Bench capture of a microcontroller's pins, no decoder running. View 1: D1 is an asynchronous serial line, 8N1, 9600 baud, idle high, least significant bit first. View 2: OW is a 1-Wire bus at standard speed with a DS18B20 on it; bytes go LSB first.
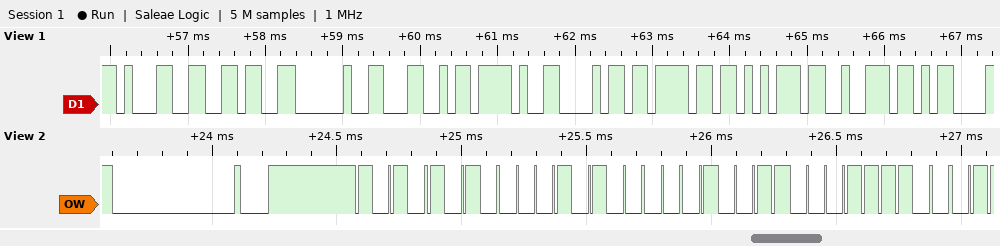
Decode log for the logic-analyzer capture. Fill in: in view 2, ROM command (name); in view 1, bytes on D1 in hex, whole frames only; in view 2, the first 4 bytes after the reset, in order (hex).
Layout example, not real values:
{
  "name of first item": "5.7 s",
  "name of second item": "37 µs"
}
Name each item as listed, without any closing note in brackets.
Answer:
{
  "in view 2, ROM command": "Match ROM",
  "in view 1, bytes on D1 in hex, whole frames only": "31 36 20 4C 2F 68 6F 75 72 0D",
  "in view 2, the first 4 bytes after the reset, in order": "55 28 C8 78"
}
